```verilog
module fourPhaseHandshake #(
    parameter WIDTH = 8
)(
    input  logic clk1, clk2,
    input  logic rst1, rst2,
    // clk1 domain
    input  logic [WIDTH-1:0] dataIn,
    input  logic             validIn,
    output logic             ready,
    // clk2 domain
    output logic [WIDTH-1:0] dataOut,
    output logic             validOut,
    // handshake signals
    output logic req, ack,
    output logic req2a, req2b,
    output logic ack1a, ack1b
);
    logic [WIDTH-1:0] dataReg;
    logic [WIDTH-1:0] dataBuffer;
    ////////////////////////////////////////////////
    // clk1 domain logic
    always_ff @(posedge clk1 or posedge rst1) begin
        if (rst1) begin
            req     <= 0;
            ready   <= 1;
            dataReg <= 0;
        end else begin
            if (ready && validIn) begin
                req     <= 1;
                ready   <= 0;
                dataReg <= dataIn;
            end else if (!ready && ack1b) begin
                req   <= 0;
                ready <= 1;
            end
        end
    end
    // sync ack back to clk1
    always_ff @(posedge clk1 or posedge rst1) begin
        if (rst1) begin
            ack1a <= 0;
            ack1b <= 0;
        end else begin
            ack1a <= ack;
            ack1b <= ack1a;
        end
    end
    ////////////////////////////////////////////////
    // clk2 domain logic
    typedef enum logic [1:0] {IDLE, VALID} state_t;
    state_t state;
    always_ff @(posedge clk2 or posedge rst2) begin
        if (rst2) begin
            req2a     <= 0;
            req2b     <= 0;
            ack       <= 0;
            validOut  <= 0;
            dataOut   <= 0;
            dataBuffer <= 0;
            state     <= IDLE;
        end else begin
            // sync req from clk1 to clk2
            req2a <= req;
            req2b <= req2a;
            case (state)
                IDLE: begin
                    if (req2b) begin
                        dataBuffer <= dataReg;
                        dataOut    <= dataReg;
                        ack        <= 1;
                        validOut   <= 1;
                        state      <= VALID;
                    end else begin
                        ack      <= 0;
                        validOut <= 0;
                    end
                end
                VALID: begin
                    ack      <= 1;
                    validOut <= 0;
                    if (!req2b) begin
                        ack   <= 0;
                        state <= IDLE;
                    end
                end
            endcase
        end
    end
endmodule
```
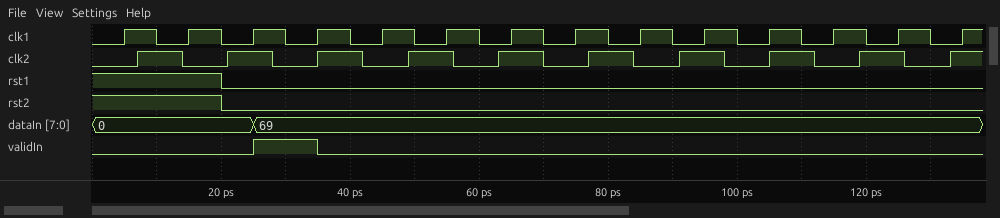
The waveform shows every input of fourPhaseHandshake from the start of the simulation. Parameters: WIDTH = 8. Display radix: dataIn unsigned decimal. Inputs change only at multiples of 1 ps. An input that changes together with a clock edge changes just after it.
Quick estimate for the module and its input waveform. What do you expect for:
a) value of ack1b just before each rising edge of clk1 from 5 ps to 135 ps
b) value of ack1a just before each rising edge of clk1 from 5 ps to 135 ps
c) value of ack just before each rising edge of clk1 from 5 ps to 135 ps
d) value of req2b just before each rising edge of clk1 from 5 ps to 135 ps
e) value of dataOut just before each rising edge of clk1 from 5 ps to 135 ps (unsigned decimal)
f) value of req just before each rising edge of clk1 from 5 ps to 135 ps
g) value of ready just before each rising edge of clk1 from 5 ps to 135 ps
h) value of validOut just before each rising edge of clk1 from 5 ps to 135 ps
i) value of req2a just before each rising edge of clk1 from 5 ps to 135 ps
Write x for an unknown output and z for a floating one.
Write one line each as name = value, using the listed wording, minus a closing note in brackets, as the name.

value of ack1b just before each rising edge of clk1 from 5 ps to 135 ps = 0 0 0 0 0 0 0 0 0 0 1 1 1 1
value of ack1a just before each rising edge of clk1 from 5 ps to 135 ps = 0 0 0 0 0 0 0 0 0 1 1 1 1 1
value of ack just before each rising edge of clk1 from 5 ps to 135 ps = 0 0 0 0 0 0 0 0 1 1 1 1 1 1
value of req2b just before each rising edge of clk1 from 5 ps to 135 ps = 0 0 0 0 0 0 1 1 1 1 1 1 1 0
value of dataOut just before each rising edge of clk1 from 5 ps to 135 ps = 0, 0, 0, 0, 0, 0, 0, 0, 69, 69, 69, 69, 69, 69
value of req just before each rising edge of clk1 from 5 ps to 135 ps = 0 0 0 0 1 1 1 1 1 1 1 0 0 0
value of ready just before each rising edge of clk1 from 5 ps to 135 ps = 1 1 1 1 0 0 0 0 0 0 0 1 1 1
value of validOut just before each rising edge of clk1 from 5 ps to 135 ps = 0 0 0 0 0 0 0 0 1 0 0 0 0 0
value of req2a just before each rising edge of clk1 from 5 ps to 135 ps = 0 0 0 0 0 1 1 1 1 1 1 1 0 0
